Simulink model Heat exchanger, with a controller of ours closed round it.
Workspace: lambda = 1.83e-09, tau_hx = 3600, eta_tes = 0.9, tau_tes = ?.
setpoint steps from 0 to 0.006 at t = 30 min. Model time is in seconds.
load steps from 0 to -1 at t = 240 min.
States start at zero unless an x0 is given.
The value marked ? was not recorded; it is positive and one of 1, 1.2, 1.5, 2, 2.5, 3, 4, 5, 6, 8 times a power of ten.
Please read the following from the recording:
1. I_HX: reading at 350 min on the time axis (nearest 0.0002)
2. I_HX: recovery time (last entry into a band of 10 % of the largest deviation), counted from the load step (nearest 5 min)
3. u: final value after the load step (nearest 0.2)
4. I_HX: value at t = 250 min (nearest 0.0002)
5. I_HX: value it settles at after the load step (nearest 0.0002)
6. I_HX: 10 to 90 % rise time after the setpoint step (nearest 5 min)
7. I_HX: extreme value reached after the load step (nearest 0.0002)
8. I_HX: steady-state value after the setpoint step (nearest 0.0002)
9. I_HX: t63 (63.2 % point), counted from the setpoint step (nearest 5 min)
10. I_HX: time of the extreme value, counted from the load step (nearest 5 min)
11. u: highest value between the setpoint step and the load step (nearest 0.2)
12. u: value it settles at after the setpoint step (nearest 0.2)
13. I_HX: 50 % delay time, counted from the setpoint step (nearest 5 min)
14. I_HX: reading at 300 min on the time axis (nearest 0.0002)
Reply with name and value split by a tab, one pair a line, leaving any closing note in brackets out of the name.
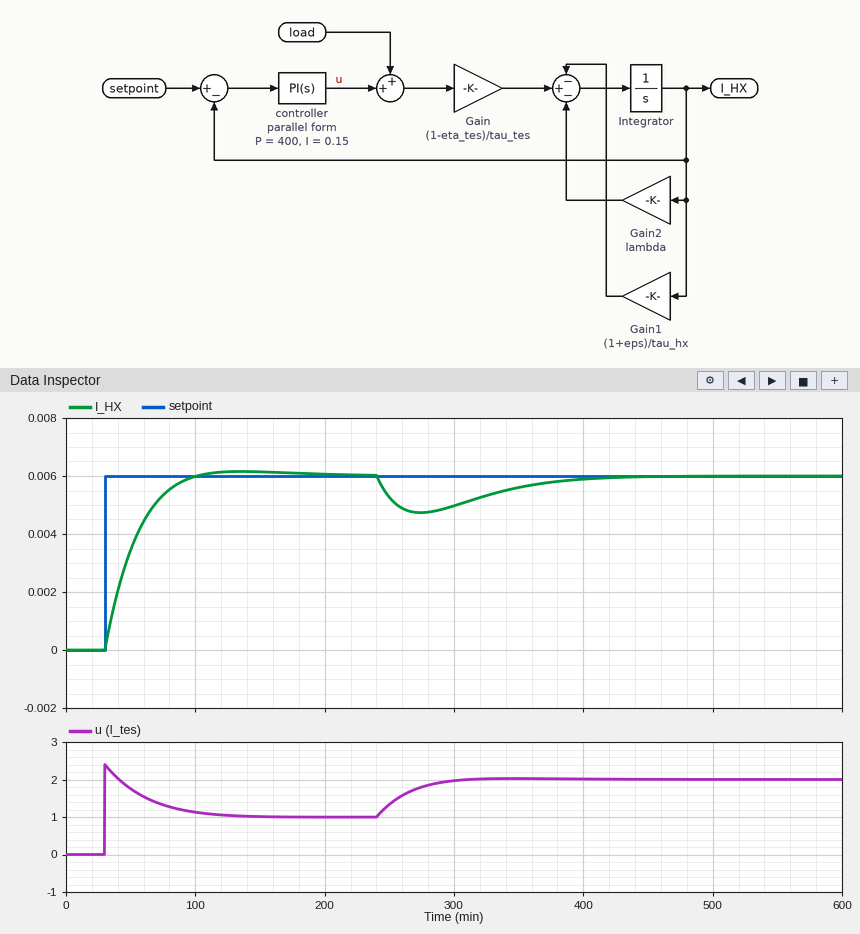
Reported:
I_HX: reading at 350 min on the time axis	0.0056
I_HX: recovery time (last entry into a band of 10 % of the largest deviation), counted from the load step	155 min
u: final value after the load step	2.0
I_HX: value at t = 250 min	0.0052
I_HX: value it settles at after the load step	0.0060
I_HX: 10 to 90 % rise time after the setpoint step	45 min
I_HX: extreme value reached after the load step	0.0048
I_HX: steady-state value after the setpoint step	0.0060
I_HX: t63 (63.2 % point), counted from the setpoint step	25 min
I_HX: time of the extreme value, counted from the load step	35 min
u: highest value between the setpoint step and the load step	2.4
u: value it settles at after the setpoint step	1.0
I_HX: 50 % delay time, counted from the setpoint step	15 min
I_HX: reading at 300 min on the time axis	0.0050
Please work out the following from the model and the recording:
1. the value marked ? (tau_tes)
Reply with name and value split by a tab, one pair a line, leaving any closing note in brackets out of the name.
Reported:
the value marked ?	60000
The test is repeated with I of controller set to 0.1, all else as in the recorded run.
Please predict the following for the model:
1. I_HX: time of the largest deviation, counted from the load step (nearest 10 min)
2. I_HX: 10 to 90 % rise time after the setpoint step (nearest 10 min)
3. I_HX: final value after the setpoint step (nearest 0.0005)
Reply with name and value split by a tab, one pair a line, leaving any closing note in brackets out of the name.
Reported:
I_HX: time of the largest deviation, counted from the load step	40 min
I_HX: 10 to 90 % rise time after the setpoint step	60 min
I_HX: final value after the setpoint step	0.0060
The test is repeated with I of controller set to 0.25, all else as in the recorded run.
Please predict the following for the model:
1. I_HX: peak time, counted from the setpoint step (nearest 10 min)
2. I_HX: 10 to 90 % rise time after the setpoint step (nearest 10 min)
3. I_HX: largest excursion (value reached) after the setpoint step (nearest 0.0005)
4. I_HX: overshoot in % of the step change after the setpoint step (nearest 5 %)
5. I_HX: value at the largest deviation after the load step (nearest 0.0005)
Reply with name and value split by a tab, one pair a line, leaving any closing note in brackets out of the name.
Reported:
I_HX: peak time, counted from the setpoint step	70 min
I_HX: 10 to 90 % rise time after the setpoint step	30 min
I_HX: largest excursion (value reached) after the setpoint step	0.0065
I_HX: overshoot in % of the step change after the setpoint step	10 %
I_HX: value at the largest deviation after the load step	0.0050
